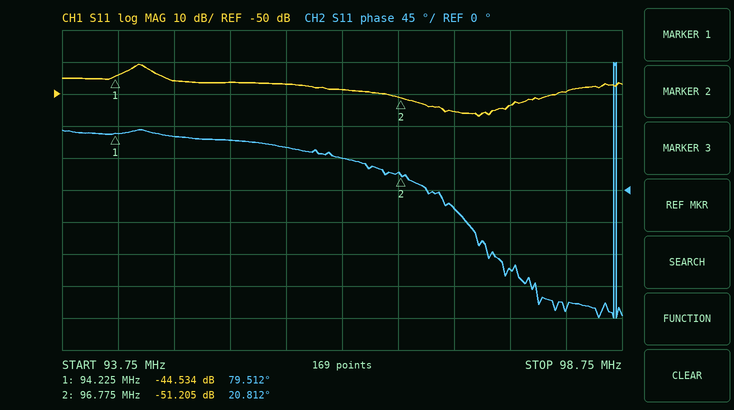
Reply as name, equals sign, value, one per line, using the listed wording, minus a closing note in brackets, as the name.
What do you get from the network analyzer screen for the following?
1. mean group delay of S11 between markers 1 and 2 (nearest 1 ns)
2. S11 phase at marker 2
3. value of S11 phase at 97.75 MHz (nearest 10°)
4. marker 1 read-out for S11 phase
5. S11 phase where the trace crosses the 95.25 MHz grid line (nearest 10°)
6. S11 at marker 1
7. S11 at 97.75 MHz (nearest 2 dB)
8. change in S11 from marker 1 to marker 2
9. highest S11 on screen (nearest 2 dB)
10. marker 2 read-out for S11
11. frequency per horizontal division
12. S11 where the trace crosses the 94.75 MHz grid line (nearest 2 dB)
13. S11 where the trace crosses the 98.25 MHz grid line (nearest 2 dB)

mean group delay of S11 between markers 1 and 2 = 64 ns
S11 phase at marker 2 = 20.812°
value of S11 phase at 97.75 MHz = -110°
marker 1 read-out for S11 phase = 79.512°
S11 phase where the trace crosses the 95.25 MHz grid line = 70°
S11 at marker 1 = -44.534 dB
S11 at 97.75 MHz = -54 dB
change in S11 from marker 1 to marker 2 = -6.671 dB
highest S11 on screen = -40 dB
marker 2 read-out for S11 = -51.205 dB
frequency per horizontal division = 500 kHz
S11 where the trace crosses the 94.75 MHz grid line = -46 dB
S11 where the trace crosses the 98.25 MHz grid line = -50 dB
